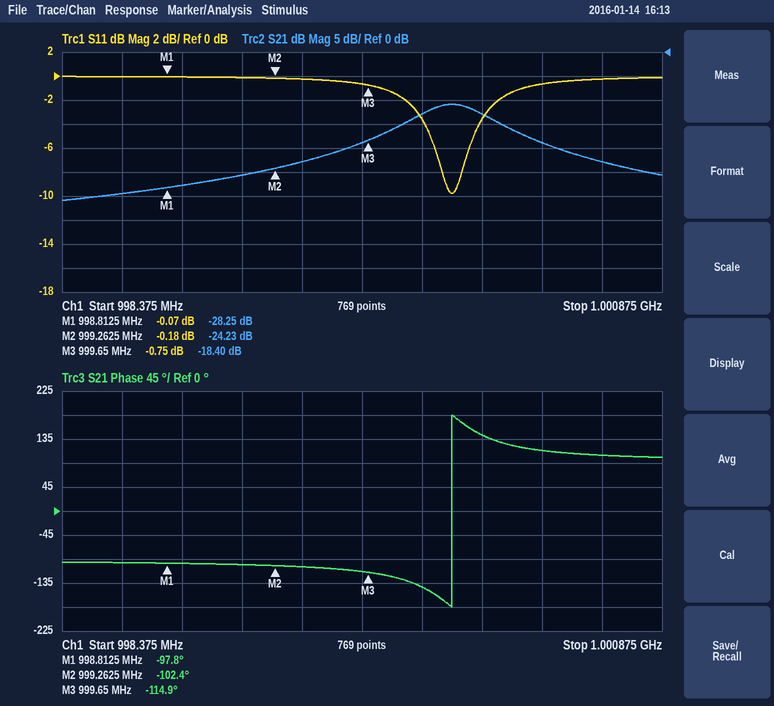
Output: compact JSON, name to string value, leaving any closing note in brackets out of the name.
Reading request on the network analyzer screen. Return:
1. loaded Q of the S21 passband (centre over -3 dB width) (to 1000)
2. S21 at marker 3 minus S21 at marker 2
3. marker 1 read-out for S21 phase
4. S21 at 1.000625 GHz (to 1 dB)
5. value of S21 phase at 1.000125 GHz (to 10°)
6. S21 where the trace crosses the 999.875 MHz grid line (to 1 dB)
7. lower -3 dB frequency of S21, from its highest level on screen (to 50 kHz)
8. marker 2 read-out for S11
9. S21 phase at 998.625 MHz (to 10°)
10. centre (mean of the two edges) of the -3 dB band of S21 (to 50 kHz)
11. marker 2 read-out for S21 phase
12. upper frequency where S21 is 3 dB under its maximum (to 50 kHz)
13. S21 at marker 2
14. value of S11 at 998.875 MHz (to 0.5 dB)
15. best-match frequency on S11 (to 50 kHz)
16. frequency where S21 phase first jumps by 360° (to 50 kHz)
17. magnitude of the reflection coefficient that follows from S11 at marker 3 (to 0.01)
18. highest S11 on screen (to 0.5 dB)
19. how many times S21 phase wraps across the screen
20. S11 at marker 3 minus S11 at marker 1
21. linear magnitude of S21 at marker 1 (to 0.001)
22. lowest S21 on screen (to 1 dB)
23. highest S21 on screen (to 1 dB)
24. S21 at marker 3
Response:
{"loaded Q of the S21 passband (centre over -3 dB width)": "3000", "S21 at marker 3 minus S21 at marker 2": "5.83 dB", "marker 1 read-out for S21 phase": "-97.8°", "S21 at 1.000625 GHz": "-23 dB", "value of S21 phase at 1.000125 GHz": "140°", "S21 where the trace crosses the 999.875 MHz grid line": "-13 dB", "lower -3 dB frequency of S21, from its highest level on screen": "999.85 MHz", "marker 2 read-out for S11": "-0.18 dB", "S21 phase at 998.625 MHz": "-100°", "centre (mean of the two edges) of the -3 dB band of S21": "1.00000 GHz", "marker 2 read-out for S21 phase": "-102.4°", "upper frequency where S21 is 3 dB under its maximum": "1.00015 GHz", "S21 at marker 2": "-24.23 dB", "value of S11 at 998.875 MHz": "0.0 dB", "best-match frequency on S11": "1.00000 GHz", "frequency where S21 phase first jumps by 360°": "1.00000 GHz", "magnitude of the reflection coefficient that follows from S11 at marker 3": "0.92", "highest S11 on screen": "0.0 dB", "how many times S21 phase wraps across the screen": "1", "S11 at marker 3 minus S11 at marker 1": "-0.68 dB", "linear magnitude of S21 at marker 1": "0.039", "lowest S21 on screen": "-31 dB", "highest S21 on screen": "-11 dB", "S21 at marker 3": "-18.40 dB"}
